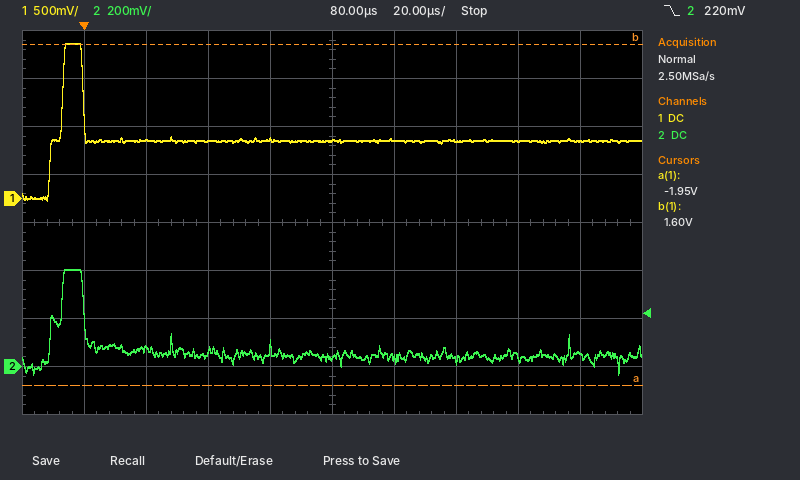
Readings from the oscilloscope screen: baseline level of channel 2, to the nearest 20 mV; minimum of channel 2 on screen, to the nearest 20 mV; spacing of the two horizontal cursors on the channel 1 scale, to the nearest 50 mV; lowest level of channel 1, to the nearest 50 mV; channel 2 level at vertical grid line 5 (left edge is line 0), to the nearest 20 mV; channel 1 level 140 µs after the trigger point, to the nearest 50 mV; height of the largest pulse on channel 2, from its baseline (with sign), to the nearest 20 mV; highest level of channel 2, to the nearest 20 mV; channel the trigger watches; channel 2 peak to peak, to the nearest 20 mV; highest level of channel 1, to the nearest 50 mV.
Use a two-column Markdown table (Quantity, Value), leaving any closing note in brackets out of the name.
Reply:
| Quantity | Value |
|---|---|
| baseline level of channel 2, to the nearest 20 mV | 40 mV |
| minimum of channel 2 on screen, to the nearest 20 mV | -40 mV |
| spacing of the two horizontal cursors on the channel 1 scale, to the nearest 50 mV | 3.55 V |
| lowest level of channel 1, to the nearest 50 mV | 0 mV |
| channel 2 level at vertical grid line 5 (left edge is line 0), to the nearest 20 mV | 40 mV |
| channel 1 level 140 µs after the trigger point, to the nearest 50 mV | 600 mV |
| height of the largest pulse on channel 2, from its baseline (with sign), to the nearest 20 mV | +360 mV |
| highest level of channel 2, to the nearest 20 mV | 400 mV |
| channel the trigger watches | channel 2 |
| channel 2 peak to peak, to the nearest 20 mV | 440 mV |
| highest level of channel 1, to the nearest 50 mV | 1.60 V |
